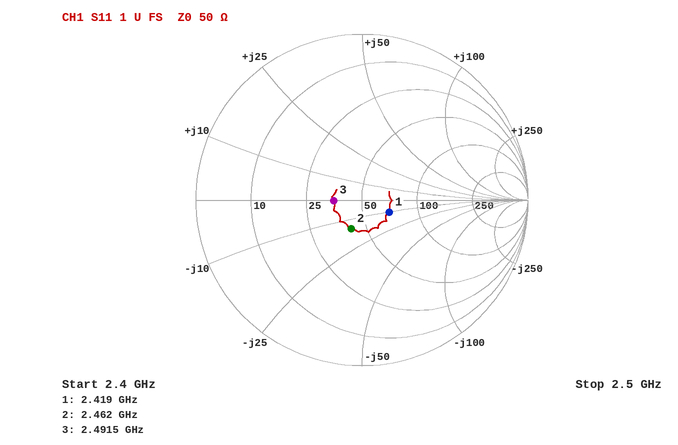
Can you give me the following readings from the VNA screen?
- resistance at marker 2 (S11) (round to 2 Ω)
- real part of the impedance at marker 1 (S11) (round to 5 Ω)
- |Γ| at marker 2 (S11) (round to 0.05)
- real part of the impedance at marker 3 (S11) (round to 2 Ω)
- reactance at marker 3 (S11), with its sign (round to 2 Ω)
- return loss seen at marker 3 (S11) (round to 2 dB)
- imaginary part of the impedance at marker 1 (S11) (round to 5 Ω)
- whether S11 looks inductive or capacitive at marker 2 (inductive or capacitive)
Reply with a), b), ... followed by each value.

a) 42 Ω
b) 70 Ω
c) 0.20
d) 36 Ω
e) 0 Ω
f) 16 dB
g) -10 Ω
h) capacitive
